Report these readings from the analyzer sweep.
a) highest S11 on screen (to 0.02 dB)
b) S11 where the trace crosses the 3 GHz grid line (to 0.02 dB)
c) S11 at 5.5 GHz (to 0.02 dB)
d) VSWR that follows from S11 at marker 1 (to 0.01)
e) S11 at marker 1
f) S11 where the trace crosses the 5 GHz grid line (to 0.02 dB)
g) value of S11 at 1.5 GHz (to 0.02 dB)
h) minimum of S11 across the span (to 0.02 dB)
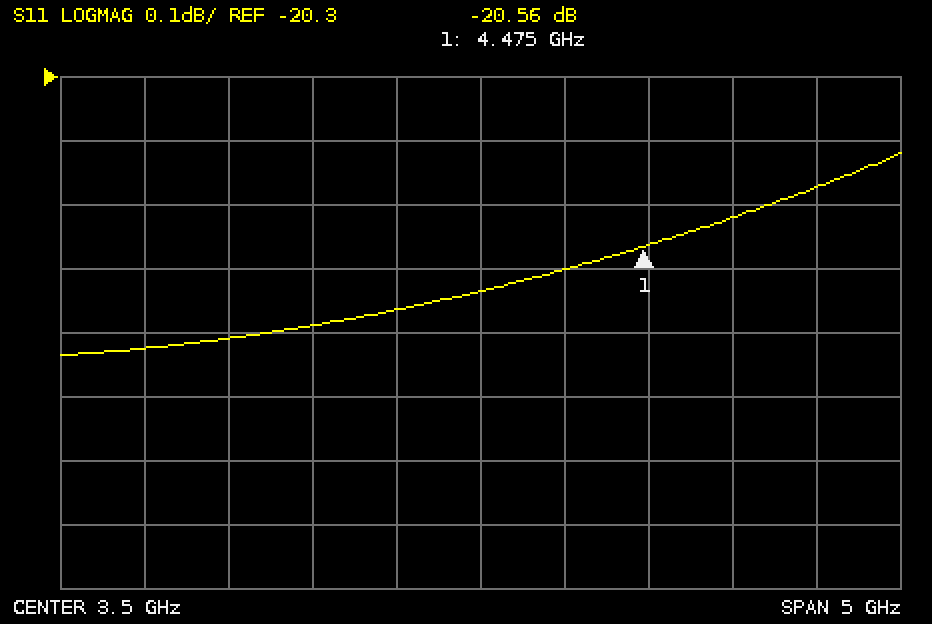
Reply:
-20.42 dB
-20.66 dB
-20.48 dB
1.21
-20.56 dB
-20.52 dB
-20.72 dB
-20.74 dB
